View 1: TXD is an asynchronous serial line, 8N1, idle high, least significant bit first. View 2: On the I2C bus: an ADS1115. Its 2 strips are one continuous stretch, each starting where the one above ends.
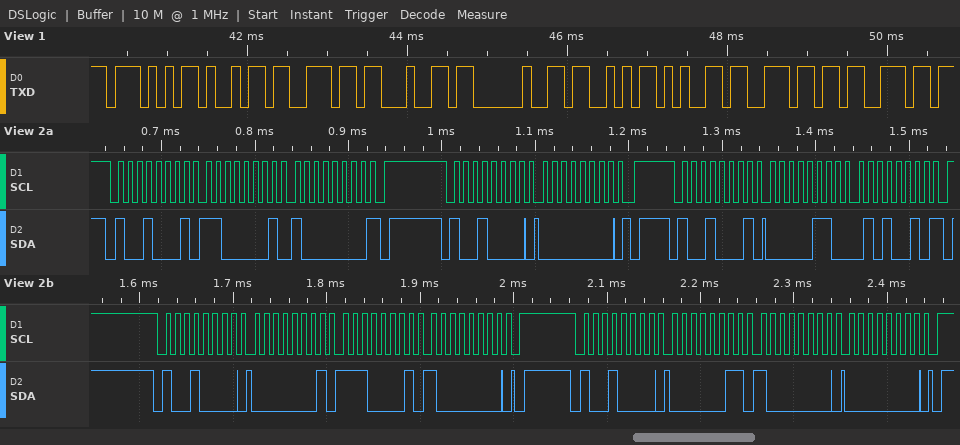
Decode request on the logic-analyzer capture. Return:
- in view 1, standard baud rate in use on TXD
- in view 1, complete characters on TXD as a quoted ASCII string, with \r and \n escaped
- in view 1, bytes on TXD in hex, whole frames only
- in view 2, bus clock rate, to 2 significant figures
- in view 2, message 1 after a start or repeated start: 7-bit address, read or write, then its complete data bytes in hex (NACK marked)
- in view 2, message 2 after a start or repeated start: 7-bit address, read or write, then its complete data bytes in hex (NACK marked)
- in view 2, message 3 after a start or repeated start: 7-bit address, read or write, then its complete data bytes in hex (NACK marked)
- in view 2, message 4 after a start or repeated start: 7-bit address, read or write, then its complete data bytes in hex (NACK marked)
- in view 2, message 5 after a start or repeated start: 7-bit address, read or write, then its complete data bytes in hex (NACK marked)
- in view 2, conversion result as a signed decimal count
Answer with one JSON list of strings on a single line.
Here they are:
["9600 baud", "\"Wind Sens\"", "57 69 6E 64 20 53 65 6E 73", "100 kHz", "0x48 read: C1 80 NACK", "0x48 write: 00", "0x48 read: 06 52 NACK", "0x48 write: 01 E1 80", "0x48 write: 03 80 00", "1618"]
